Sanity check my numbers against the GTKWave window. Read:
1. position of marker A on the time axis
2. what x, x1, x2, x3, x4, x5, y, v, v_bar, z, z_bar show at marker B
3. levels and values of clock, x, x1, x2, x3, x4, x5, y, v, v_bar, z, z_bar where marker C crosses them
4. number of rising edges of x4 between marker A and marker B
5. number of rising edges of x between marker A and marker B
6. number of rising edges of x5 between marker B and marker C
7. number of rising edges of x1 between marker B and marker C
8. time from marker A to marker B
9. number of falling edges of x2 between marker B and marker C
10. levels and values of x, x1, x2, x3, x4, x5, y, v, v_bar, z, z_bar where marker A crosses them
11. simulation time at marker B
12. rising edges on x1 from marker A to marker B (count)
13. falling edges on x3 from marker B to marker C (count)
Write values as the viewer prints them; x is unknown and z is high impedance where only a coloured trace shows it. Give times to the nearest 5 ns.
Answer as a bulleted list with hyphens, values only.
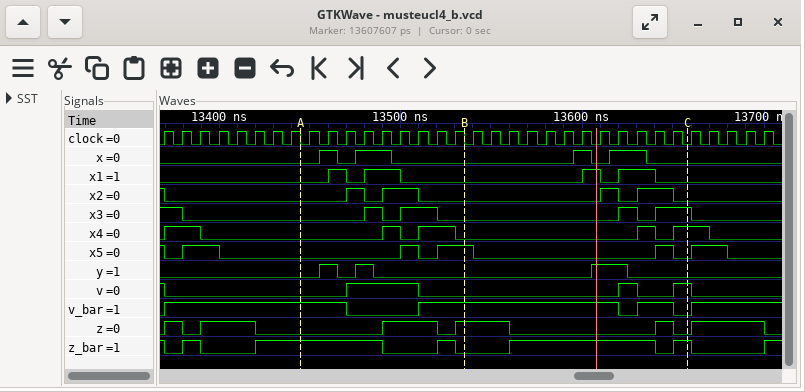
- 13445 ns
- x=0, x1=0, x2=0, x3=0, x4=0, x5=1, y=0, v=0, v_bar=1, z=1, z_bar=0
- clock=0, x=0, x1=0, x2=0, x3=1, x4=1, x5=0, y=0, v=1, v_bar=0, z=0, z_bar=1
- 2
- 2
- 1
- 2
- 90 ns
- 2
- x=0, x1=0, x2=0, x3=0, x4=0, x5=0, y=0, v=0, v_bar=1, z=0, z_bar=1
- 13535 ns
- 2
- 1
